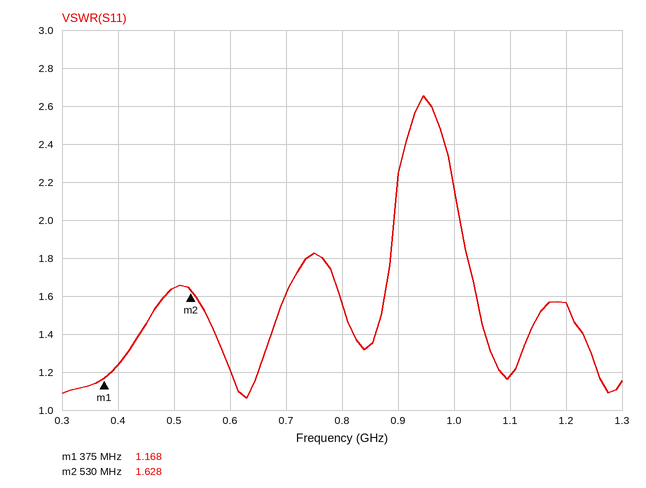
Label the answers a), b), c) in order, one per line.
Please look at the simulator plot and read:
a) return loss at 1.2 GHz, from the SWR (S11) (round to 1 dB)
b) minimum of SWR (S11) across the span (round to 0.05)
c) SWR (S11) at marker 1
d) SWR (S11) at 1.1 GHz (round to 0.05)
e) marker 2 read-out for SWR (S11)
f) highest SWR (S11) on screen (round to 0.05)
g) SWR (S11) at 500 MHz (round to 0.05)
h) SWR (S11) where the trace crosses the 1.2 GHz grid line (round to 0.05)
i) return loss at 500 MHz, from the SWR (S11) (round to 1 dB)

a) 13 dB
b) 1.05
c) 1.168
d) 1.20
e) 1.628
f) 2.65
g) 1.65
h) 1.55
i) 12 dB
